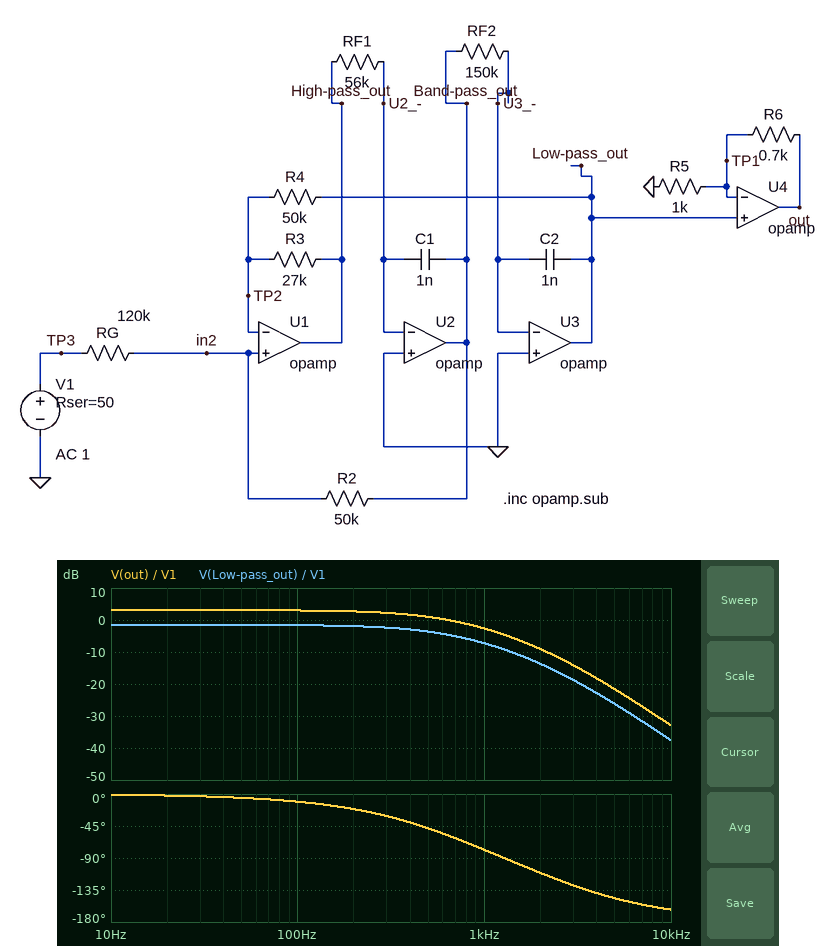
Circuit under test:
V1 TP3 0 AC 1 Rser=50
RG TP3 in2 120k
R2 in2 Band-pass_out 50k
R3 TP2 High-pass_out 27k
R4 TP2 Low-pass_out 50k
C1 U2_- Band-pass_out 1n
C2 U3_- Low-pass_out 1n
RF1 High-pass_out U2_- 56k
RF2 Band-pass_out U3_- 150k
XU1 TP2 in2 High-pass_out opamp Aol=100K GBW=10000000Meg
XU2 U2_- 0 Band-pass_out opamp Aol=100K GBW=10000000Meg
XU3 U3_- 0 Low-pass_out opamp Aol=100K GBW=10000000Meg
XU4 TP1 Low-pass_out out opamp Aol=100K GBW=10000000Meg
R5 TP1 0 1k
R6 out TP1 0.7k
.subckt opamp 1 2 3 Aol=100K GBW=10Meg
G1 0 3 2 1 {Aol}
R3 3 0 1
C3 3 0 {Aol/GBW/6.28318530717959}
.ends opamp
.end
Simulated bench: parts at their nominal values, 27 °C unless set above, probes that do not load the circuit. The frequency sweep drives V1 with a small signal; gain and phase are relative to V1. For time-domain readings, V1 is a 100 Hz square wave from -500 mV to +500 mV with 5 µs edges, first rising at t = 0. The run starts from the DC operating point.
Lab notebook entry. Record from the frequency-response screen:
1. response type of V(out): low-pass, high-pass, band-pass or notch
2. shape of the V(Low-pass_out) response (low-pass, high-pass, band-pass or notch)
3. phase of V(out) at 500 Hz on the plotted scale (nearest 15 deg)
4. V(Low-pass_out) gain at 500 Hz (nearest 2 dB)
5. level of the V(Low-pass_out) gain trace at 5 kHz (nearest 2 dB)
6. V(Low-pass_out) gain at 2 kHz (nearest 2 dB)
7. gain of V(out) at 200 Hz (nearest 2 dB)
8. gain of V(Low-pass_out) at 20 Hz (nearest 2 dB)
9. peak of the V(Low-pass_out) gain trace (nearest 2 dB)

low-pass
low-pass
-45 deg
-4 dB
-26 dB
-14 dB
2 dB
-2 dB
-2 dB
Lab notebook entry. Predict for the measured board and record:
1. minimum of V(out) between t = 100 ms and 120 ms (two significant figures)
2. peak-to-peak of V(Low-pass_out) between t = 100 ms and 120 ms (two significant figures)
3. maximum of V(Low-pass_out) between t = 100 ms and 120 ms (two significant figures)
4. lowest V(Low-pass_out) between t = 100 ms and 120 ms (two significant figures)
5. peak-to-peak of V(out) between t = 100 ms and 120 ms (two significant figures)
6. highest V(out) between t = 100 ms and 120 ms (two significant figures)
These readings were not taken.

-710 mV
840 mV
420 mV
-420 mV
1.4 V
710 mV
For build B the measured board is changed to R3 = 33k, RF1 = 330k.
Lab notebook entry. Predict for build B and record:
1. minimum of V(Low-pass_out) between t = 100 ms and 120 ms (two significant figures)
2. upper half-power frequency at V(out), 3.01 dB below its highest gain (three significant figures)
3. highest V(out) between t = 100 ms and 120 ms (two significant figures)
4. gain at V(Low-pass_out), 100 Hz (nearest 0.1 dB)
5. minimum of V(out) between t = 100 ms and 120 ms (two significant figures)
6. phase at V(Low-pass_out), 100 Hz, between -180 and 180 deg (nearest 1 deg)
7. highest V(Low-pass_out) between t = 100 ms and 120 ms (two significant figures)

-500 mV
682 Hz
850 mV
-2.5 dB
-850 mV
-10 deg
500 mV
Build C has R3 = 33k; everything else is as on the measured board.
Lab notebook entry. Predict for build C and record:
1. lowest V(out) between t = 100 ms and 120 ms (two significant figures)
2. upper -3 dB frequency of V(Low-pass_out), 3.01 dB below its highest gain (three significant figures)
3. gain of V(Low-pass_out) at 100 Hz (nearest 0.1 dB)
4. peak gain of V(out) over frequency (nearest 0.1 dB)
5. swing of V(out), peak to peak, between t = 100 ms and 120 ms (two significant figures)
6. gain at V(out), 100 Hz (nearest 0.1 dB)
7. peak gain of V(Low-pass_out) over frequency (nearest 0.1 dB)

-630 mV
720 Hz
-2.7 dB
2.0 dB
1.3 V
1.9 dB
-2.6 dB
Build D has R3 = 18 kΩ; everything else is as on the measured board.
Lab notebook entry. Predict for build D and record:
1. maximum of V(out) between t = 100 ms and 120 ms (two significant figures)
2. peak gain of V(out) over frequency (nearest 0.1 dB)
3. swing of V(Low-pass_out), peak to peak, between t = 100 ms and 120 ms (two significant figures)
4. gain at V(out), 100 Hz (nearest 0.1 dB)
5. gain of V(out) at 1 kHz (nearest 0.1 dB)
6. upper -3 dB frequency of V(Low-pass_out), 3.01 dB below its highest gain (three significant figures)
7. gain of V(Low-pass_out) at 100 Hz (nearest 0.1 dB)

940 mV
5.5 dB
1.1 V
5.3 dB
-2.5 dB
463 Hz
0.7 dB
